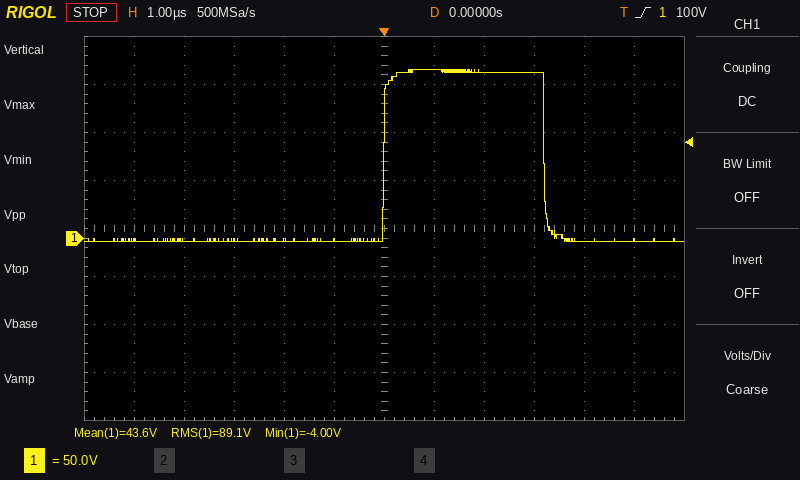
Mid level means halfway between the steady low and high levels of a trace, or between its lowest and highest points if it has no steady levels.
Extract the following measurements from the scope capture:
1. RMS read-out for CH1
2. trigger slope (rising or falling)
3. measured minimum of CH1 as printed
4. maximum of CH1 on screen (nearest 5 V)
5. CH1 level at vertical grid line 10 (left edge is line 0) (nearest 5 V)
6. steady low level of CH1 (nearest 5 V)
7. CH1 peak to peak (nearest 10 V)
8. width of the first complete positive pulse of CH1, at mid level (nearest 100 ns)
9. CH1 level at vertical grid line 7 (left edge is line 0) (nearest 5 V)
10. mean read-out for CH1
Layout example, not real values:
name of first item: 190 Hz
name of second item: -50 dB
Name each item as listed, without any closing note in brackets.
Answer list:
RMS read-out for CH1: 89.1 V
trigger slope: rising
measured minimum of CH1 as printed: -4.00 V
maximum of CH1 on screen: 175 V
CH1 level at vertical grid line 10 (left edge is line 0): -5 V
steady low level of CH1: -5 V
CH1 peak to peak: 180 V
width of the first complete positive pulse of CH1, at mid level: 3.2 µs
CH1 level at vertical grid line 7 (left edge is line 0): 175 V
mean read-out for CH1: 43.6 V
